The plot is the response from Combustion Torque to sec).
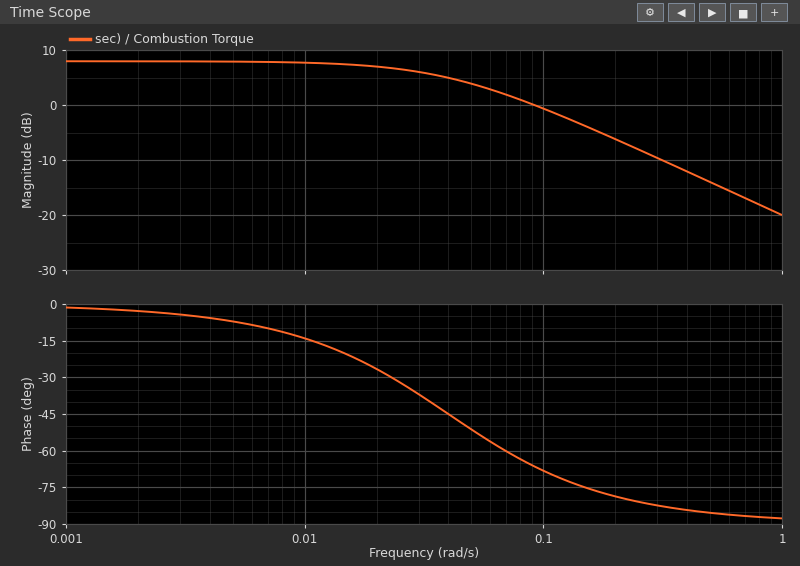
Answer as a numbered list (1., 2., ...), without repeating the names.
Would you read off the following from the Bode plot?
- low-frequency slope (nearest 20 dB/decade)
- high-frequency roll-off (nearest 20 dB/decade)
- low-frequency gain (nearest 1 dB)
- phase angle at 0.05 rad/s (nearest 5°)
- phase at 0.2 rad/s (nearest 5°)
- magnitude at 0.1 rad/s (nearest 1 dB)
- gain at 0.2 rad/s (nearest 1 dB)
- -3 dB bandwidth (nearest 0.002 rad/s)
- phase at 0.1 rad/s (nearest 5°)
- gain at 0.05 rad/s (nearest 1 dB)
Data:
1. 0 dB/decade
2. -20 dB/decade
3. 8 dB
4. -50°
5. -80°
6. -1 dB
7. -6 dB
8. 0.040 rad/s
9. -70°
10. 4 dB
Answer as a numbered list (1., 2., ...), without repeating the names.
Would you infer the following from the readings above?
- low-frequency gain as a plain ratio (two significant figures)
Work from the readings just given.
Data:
1. 2.5
